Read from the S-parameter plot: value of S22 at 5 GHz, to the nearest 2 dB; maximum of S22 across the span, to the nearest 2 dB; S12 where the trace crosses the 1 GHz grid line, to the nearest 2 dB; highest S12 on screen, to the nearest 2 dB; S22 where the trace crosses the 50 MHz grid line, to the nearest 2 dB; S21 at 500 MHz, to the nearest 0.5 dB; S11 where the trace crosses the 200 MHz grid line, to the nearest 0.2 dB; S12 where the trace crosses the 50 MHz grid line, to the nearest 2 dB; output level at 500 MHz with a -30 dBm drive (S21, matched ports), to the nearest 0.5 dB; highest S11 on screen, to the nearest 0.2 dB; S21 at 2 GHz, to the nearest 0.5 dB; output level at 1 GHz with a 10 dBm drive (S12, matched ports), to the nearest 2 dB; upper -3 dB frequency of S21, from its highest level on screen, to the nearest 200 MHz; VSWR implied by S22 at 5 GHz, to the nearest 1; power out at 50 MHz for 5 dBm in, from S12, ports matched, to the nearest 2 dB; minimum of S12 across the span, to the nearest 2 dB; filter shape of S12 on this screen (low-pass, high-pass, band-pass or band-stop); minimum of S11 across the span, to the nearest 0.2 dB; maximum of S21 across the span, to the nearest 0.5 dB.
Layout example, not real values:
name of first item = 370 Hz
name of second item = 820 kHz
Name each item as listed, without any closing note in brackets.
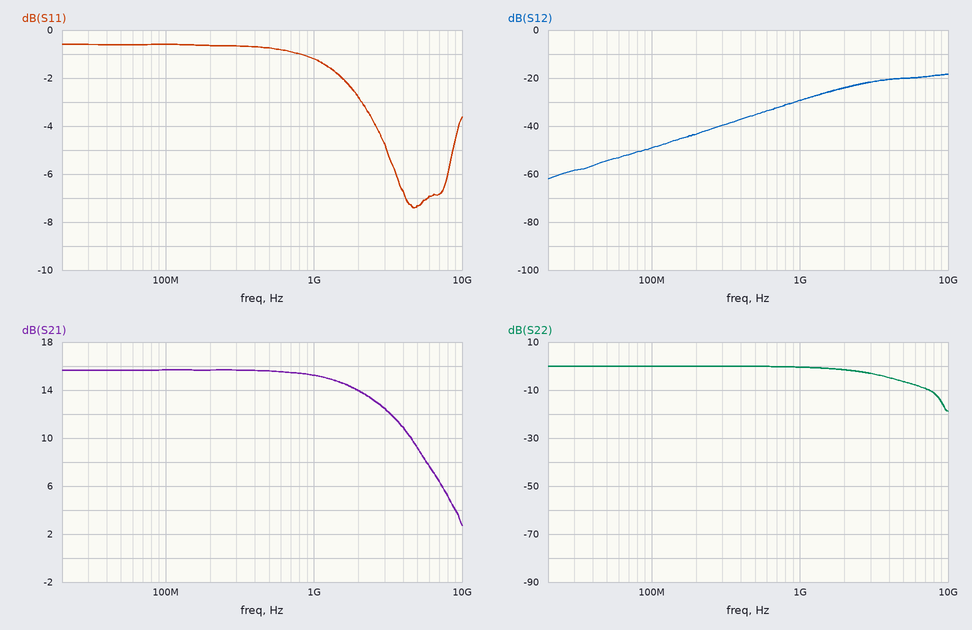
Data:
value of S22 at 5 GHz, to the nearest 2 dB = -6 dB
maximum of S22 across the span, to the nearest 2 dB = 0 dB
S12 where the trace crosses the 1 GHz grid line, to the nearest 2 dB = -30 dB
highest S12 on screen, to the nearest 2 dB = -18 dB
S22 where the trace crosses the 50 MHz grid line, to the nearest 2 dB = 0 dB
S21 at 500 MHz, to the nearest 0.5 dB = 15.5 dB
S11 where the trace crosses the 200 MHz grid line, to the nearest 0.2 dB = -0.6 dB
S12 where the trace crosses the 50 MHz grid line, to the nearest 2 dB = -54 dB
output level at 500 MHz with a -30 dBm drive (S21, matched ports), to the nearest 0.5 dB = -14.5 dBm
highest S11 on screen, to the nearest 0.2 dB = -0.6 dB
S21 at 2 GHz, to the nearest 0.5 dB = 14.0 dB
output level at 1 GHz with a 10 dBm drive (S12, matched ports), to the nearest 2 dB = -20 dBm
upper -3 dB frequency of S21, from its highest level on screen, to the nearest 200 MHz = 2.8 GHz
VSWR implied by S22 at 5 GHz, to the nearest 1 = 3
power out at 50 MHz for 5 dBm in, from S12, ports matched, to the nearest 2 dB = -50 dBm
minimum of S12 across the span, to the nearest 2 dB = -62 dB
filter shape of S12 on this screen = high-pass
minimum of S11 across the span, to the nearest 0.2 dB = -7.4 dB
maximum of S21 across the span, to the nearest 0.5 dB = 15.5 dB
